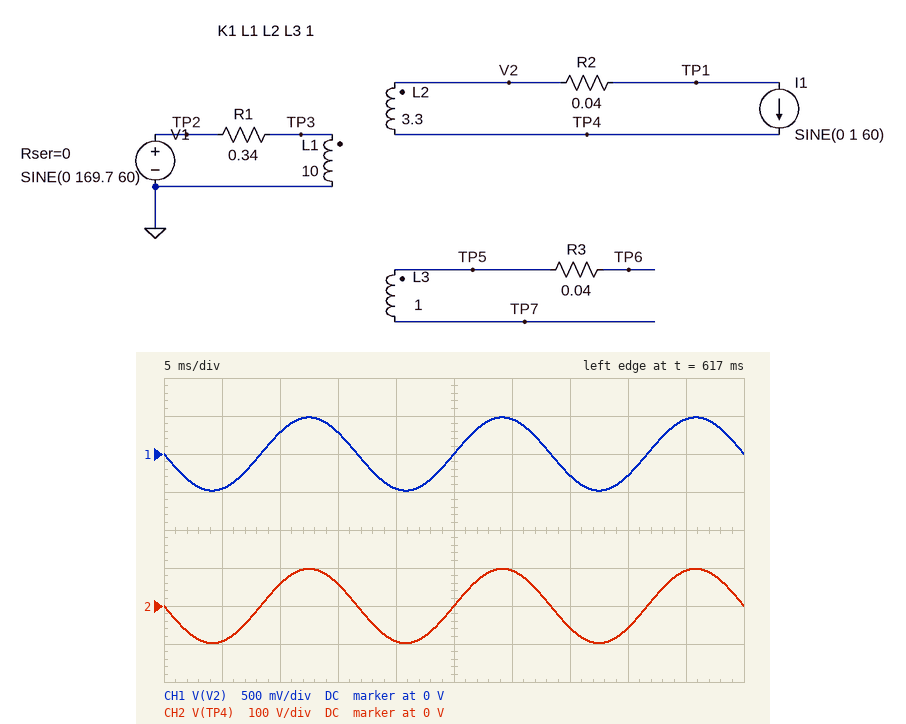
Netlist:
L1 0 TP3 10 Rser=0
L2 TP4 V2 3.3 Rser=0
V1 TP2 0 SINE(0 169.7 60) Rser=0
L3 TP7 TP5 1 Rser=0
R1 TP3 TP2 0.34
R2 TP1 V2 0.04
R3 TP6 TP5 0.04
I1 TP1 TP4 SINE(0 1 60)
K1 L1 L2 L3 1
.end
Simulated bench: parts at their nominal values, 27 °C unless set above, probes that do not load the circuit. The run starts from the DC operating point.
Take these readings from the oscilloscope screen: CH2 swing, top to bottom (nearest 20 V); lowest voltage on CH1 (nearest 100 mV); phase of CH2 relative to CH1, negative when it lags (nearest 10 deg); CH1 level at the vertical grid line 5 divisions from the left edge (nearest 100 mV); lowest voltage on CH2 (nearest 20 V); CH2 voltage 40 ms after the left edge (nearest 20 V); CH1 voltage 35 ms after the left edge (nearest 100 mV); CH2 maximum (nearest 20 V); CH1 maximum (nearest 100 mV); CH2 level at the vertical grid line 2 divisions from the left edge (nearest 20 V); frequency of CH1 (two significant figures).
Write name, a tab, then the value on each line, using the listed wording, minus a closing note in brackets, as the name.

CH2 swing, top to bottom	200 V
lowest voltage on CH1	-500 mV
phase of CH2 relative to CH1, negative when it lags	0 deg
CH1 level at the vertical grid line 5 divisions from the left edge	0 V
lowest voltage on CH2	-100 V
CH2 voltage 40 ms after the left edge	-60 V
CH1 voltage 35 ms after the left edge	-300 mV
CH2 maximum	100 V
CH1 maximum	500 mV
CH2 level at the vertical grid line 2 divisions from the left edge	60 V
frequency of CH1	60 Hz
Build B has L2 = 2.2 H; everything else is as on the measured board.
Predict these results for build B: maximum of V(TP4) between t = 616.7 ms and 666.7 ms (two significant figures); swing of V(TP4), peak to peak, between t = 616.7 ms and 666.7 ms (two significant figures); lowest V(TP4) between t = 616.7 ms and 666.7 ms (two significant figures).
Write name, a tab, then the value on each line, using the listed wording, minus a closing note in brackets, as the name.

maximum of V(TP4) between t = 616.7 ms and 666.7 ms	80 V
swing of V(TP4), peak to peak, between t = 616.7 ms and 666.7 ms	160 V
lowest V(TP4) between t = 616.7 ms and 666.7 ms	-80 V
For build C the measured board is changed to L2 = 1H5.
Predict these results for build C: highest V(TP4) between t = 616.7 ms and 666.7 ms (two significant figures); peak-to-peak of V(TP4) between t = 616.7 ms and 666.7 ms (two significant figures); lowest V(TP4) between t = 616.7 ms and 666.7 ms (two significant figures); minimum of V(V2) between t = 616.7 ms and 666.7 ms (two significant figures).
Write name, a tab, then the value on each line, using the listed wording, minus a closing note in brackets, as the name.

highest V(TP4) between t = 616.7 ms and 666.7 ms	66 V
peak-to-peak of V(TP4) between t = 616.7 ms and 666.7 ms	130 V
lowest V(TP4) between t = 616.7 ms and 666.7 ms	-66 V
minimum of V(V2) between t = 616.7 ms and 666.7 ms	-480 mV
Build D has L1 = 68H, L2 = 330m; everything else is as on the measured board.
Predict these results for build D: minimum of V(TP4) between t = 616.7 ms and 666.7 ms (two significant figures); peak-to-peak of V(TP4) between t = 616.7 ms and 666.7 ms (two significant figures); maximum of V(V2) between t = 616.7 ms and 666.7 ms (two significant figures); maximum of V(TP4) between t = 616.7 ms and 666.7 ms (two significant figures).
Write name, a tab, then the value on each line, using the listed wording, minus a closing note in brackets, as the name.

minimum of V(TP4) between t = 616.7 ms and 666.7 ms	-12 V
peak-to-peak of V(TP4) between t = 616.7 ms and 666.7 ms	25 V
maximum of V(V2) between t = 616.7 ms and 666.7 ms	480 mV
maximum of V(TP4) between t = 616.7 ms and 666.7 ms	12 V
